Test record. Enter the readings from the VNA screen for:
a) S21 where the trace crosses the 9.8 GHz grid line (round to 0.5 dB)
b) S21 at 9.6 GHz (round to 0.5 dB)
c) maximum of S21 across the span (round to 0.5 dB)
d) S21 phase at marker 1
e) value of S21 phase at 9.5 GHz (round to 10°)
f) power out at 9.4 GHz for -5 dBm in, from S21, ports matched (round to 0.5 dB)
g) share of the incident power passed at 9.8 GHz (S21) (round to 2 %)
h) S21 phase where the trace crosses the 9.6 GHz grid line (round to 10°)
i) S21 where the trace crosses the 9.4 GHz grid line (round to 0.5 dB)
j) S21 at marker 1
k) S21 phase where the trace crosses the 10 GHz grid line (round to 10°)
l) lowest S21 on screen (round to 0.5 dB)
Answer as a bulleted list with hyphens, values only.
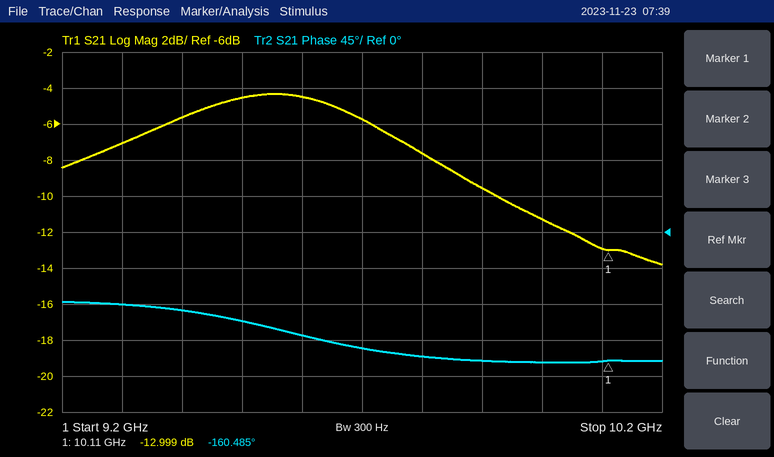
- -7.5 dB
- -4.5 dB
- -4.5 dB
- -160.485°
- -110°
- -10.5 dBm
- 18 %
- -130°
- -5.5 dB
- -12.999 dB
- -160°
- -14.0 dB
